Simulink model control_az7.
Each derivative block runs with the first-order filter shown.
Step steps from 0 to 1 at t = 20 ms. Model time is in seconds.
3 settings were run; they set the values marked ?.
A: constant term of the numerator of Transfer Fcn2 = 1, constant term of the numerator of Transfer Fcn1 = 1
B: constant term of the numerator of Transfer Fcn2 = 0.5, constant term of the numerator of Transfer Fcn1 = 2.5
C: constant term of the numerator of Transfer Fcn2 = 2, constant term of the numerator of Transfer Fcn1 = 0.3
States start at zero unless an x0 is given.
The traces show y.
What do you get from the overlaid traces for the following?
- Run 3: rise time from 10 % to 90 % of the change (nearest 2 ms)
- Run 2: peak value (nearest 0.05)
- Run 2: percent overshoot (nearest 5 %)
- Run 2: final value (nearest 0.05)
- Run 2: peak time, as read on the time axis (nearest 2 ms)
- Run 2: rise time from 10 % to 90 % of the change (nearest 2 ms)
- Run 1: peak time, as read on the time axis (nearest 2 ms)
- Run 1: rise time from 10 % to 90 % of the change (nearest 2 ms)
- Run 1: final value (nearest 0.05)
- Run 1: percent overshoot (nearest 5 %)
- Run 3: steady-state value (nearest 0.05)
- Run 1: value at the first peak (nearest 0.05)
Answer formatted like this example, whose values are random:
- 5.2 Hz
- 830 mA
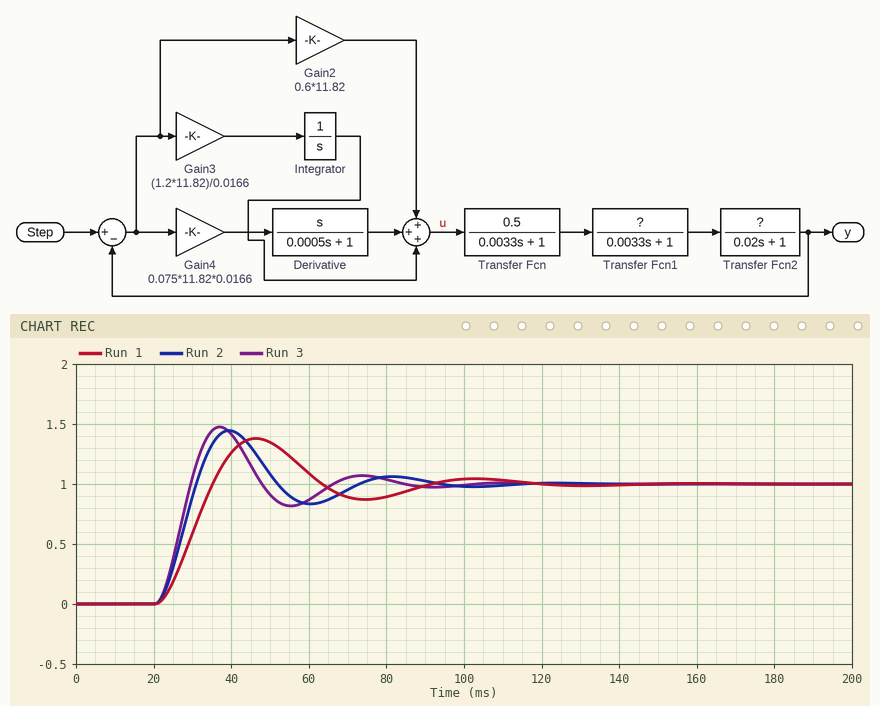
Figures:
- 6 ms
- 1.45
- 45 %
- 1.00
- 40 ms
- 8 ms
- 46 ms
- 10 ms
- 1.00
- 40 %
- 1.00
- 1.40
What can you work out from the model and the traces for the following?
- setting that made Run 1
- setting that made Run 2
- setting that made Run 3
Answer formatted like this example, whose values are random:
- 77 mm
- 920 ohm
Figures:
- C
- A
- B
